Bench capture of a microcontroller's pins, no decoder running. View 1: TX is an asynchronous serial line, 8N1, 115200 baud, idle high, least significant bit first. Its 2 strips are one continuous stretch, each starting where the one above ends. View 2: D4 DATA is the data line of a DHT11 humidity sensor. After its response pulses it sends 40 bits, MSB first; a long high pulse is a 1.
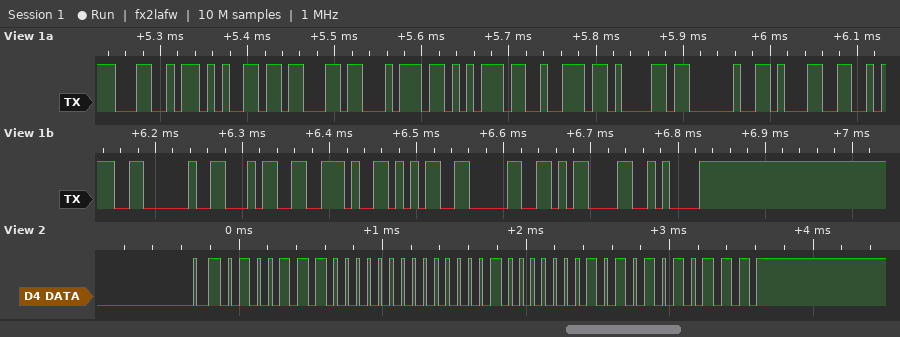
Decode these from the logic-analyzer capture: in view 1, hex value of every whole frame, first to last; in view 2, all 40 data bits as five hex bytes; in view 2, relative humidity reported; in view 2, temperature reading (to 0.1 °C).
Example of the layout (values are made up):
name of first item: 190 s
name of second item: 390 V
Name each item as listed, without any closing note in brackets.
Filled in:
in view 1, hex value of every whole frame, first to last: 4C 65 63 74 75 72 61 20 31 3A 20 34 2E 35 30 0D 0A
in view 2, all 40 data bits as five hex bytes: 4E 00 04 05 57
in view 2, relative humidity reported: 78 %
in view 2, temperature reading: 4.5 °C
